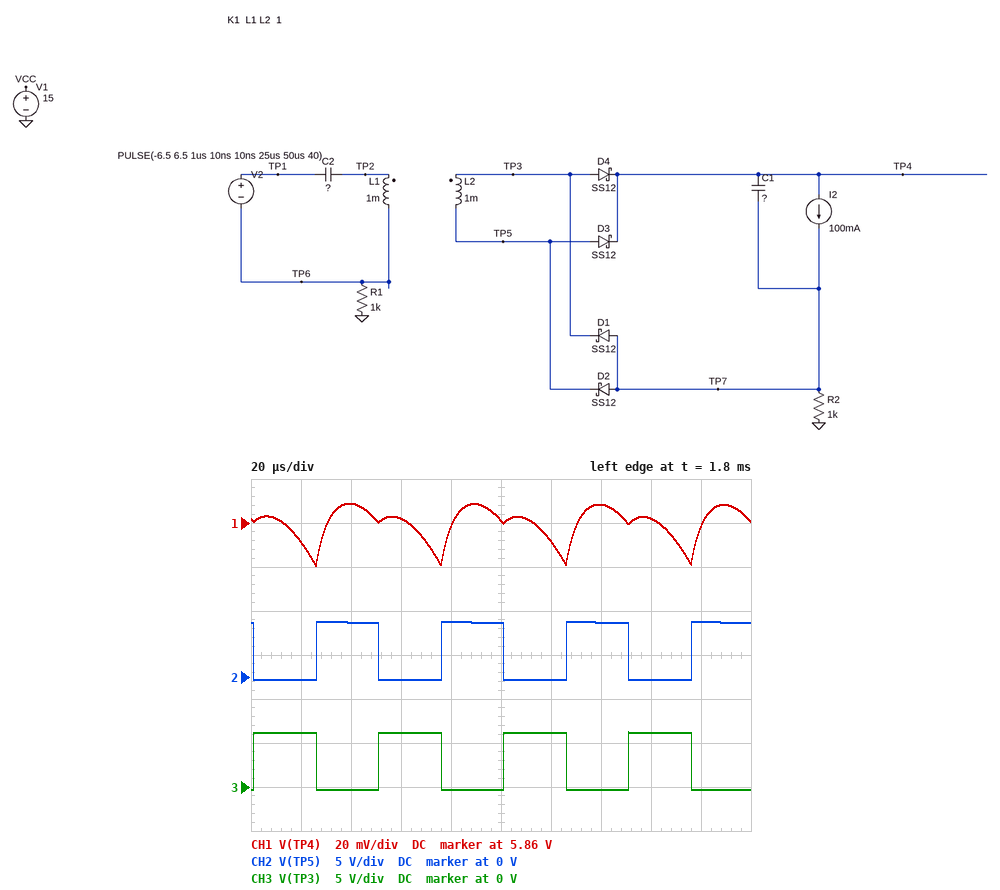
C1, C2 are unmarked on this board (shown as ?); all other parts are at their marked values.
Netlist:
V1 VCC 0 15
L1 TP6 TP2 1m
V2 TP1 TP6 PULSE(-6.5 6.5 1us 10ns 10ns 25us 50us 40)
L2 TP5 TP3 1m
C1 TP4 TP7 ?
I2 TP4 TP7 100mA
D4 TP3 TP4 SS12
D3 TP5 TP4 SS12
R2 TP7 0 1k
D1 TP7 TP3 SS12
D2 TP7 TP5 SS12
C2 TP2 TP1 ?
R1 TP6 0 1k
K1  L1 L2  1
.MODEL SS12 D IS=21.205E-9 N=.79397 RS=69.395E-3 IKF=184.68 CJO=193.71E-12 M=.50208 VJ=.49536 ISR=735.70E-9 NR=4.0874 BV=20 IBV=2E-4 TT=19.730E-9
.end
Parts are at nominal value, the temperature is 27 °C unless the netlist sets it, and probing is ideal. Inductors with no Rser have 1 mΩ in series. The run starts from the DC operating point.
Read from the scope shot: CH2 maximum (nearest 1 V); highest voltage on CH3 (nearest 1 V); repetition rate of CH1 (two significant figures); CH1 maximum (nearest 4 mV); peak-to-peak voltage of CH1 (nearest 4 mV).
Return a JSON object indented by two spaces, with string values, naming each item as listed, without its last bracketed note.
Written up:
{
  "CH2 maximum": "6 V",
  "highest voltage on CH3": "6 V",
  "repetition rate of CH1": "20 kHz",
  "CH1 maximum": "5.868 V",
  "peak-to-peak voltage of CH1": "28 mV"
}
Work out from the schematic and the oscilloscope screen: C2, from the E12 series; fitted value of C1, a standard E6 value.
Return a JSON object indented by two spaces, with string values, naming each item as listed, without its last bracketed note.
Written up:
{
  "C2, from the E12 series": "27 µF",
  "fitted value of C1, a standard E6 value": "33 µF"
}
